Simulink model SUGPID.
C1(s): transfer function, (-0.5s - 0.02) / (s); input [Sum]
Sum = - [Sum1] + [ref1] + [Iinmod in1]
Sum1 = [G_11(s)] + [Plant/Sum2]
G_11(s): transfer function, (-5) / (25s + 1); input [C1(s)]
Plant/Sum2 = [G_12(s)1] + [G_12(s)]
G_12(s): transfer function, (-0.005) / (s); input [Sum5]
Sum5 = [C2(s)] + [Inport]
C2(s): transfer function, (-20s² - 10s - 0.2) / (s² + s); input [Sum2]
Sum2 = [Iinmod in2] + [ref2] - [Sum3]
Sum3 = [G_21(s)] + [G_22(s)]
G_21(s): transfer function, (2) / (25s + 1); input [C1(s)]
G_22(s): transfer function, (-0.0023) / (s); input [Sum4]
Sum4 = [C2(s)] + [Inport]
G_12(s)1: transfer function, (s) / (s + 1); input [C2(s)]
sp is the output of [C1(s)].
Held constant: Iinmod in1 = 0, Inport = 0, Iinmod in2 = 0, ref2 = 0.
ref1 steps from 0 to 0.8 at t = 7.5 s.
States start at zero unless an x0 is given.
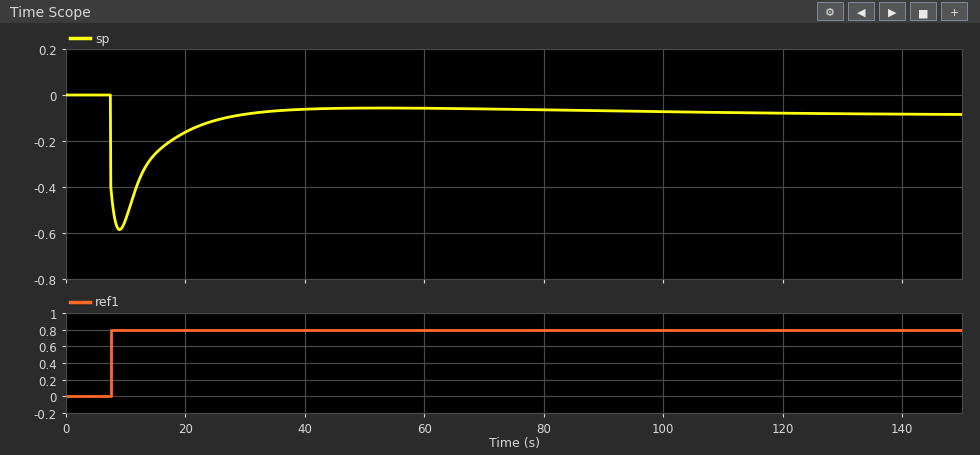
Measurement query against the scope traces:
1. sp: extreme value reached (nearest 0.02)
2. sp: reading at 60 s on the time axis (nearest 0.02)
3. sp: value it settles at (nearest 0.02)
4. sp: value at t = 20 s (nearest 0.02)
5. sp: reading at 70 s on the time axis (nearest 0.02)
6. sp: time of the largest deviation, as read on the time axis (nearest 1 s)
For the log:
-0.58
-0.06
-0.08
-0.16
-0.06
9 s
